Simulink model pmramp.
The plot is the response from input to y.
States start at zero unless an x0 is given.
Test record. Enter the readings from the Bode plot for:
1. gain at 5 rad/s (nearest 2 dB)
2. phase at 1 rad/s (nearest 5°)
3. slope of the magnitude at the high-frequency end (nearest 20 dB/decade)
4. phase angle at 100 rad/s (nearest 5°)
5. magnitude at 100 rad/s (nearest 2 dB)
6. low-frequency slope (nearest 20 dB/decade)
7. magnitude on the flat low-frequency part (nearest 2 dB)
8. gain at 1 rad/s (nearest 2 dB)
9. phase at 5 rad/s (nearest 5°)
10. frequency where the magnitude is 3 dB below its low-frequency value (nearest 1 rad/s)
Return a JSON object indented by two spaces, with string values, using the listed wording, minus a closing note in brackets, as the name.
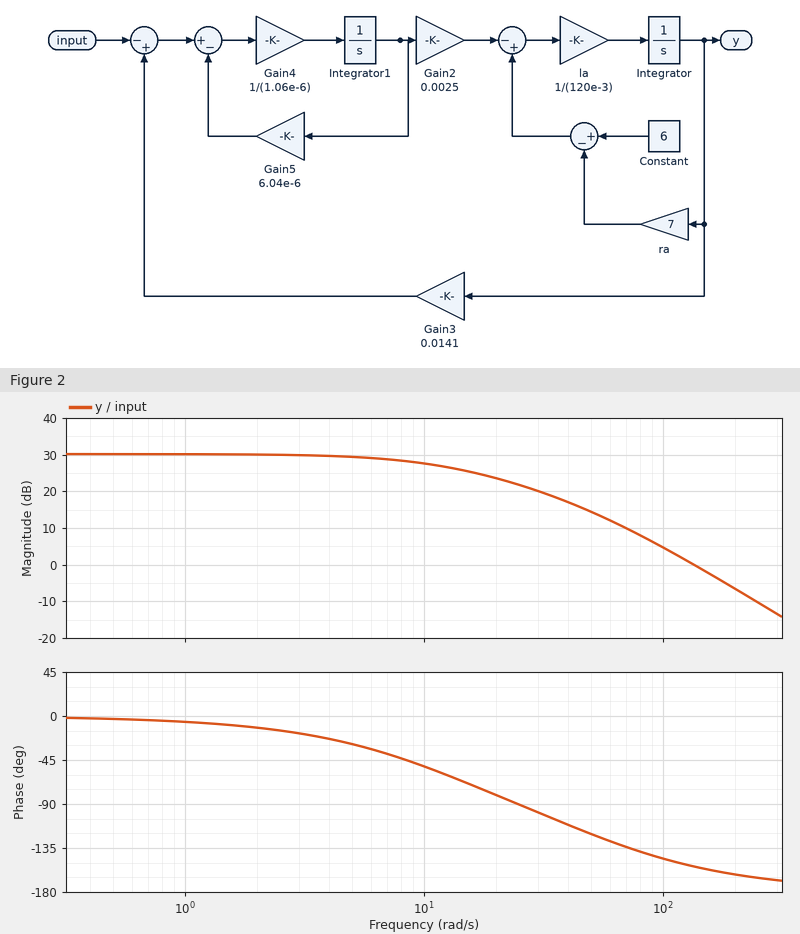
{
  "gain at 5 rad/s": "30 dB",
  "phase at 1 rad/s": "-5°",
  "slope of the magnitude at the high-frequency end": "-40 dB/decade",
  "phase angle at 100 rad/s": "-145°",
  "magnitude at 100 rad/s": "4 dB",
  "low-frequency slope": "0 dB/decade",
  "magnitude on the flat low-frequency part": "30 dB",
  "gain at 1 rad/s": "30 dB",
  "phase at 5 rad/s": "-30°",
  "frequency where the magnitude is 3 dB below its low-frequency value": "11 rad/s"
}
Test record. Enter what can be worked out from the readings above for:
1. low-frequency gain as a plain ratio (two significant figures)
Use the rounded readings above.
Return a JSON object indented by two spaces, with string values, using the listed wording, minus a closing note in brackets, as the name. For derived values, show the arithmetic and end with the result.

{
  "low-frequency gain as a plain ratio": "10^(30 / 20) = 32"
}
